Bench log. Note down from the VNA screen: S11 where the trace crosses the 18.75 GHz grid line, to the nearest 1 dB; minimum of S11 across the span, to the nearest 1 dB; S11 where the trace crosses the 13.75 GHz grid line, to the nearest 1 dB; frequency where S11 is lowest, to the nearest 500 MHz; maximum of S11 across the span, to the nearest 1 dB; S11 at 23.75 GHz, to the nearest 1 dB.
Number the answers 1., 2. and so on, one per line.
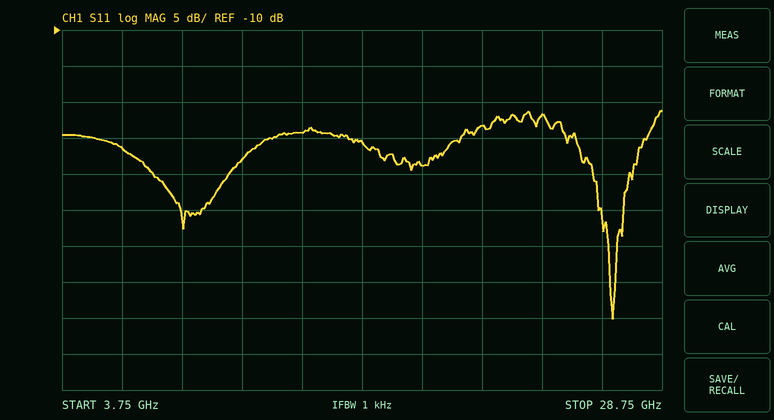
1. -29 dB
2. -50 dB
3. -24 dB
4. 26.5 GHz
5. -21 dB
6. -22 dB
